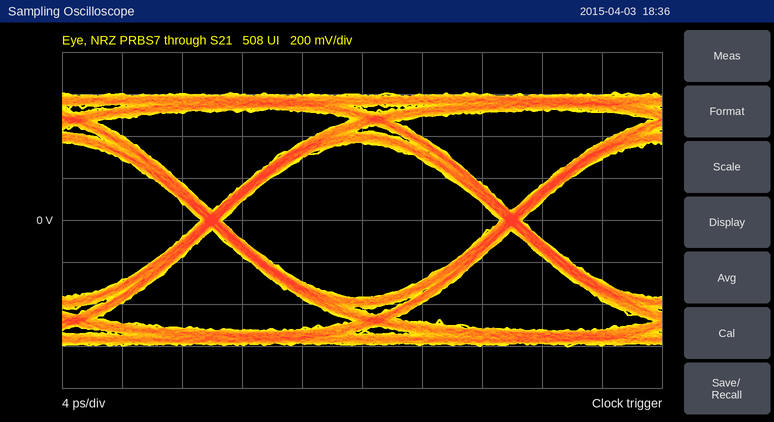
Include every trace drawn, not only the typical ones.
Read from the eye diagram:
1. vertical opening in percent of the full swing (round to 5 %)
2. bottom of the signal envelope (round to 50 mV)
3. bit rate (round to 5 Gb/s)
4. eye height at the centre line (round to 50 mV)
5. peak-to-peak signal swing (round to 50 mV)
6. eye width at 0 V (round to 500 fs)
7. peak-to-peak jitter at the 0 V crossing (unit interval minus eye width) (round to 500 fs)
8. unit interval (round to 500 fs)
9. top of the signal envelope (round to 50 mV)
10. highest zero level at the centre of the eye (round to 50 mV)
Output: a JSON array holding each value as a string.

["60 %", "-600 mV", "50 Gb/s", "750 mV", "1.20 V", "18.5 ps", "1.5 ps", "20.0 ps", "600 mV", "-350 mV"]
